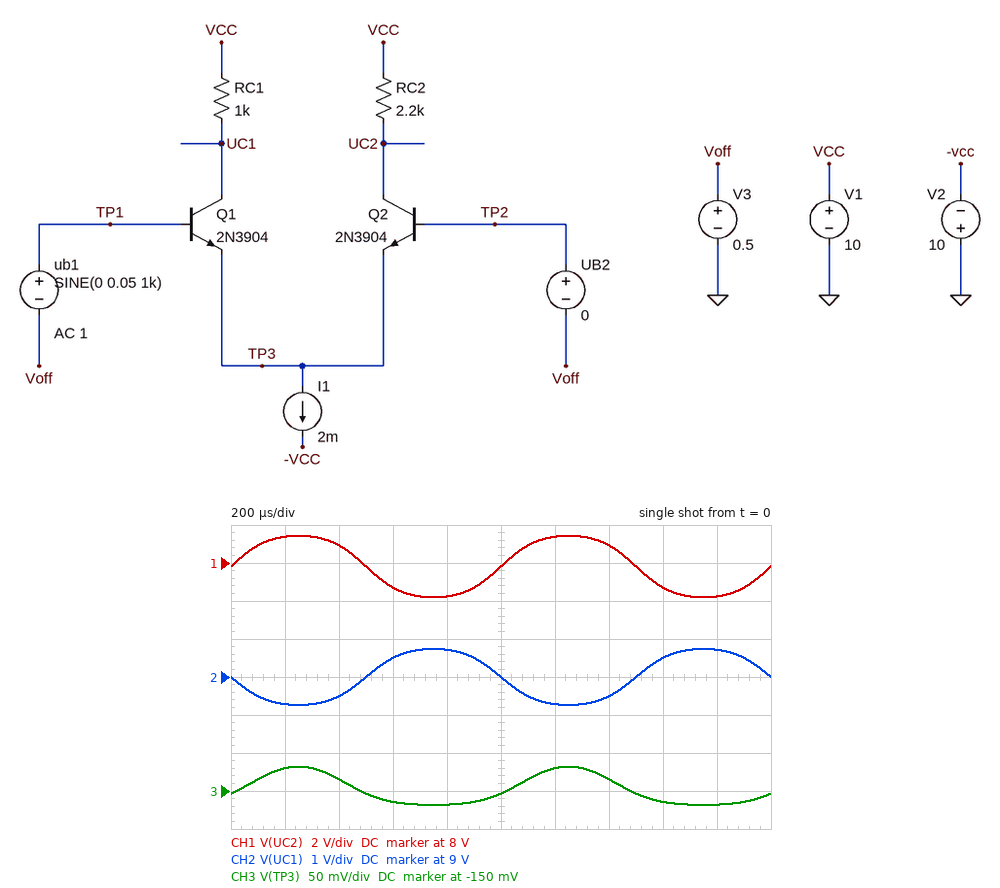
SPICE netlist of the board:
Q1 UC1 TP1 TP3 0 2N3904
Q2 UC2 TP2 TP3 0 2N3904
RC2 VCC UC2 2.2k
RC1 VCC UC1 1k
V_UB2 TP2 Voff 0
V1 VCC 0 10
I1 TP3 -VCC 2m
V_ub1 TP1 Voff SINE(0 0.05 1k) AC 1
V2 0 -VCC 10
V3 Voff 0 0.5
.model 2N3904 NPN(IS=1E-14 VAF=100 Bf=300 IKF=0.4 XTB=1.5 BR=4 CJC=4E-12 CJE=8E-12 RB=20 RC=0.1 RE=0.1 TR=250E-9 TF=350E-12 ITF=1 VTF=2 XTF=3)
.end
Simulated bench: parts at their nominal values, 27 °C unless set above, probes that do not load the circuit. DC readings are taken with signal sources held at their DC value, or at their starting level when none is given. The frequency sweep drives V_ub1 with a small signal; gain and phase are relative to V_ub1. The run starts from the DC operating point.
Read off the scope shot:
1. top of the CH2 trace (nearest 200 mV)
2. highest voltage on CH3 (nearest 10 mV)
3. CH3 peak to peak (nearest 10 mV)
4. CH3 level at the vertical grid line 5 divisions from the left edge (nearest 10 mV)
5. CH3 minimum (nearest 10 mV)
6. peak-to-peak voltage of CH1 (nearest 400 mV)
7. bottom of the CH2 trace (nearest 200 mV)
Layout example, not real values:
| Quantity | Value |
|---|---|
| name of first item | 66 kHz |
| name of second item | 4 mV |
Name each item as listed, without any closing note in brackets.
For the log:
| Quantity | Value |
|---|---|
| top of the CH2 trace | 9.8 V |
| highest voltage on CH3 | -120 mV |
| CH3 peak to peak | 50 mV |
| CH3 level at the vertical grid line 5 divisions from the left edge | -150 mV |
| CH3 minimum | -170 mV |
| peak-to-peak voltage of CH1 | 3.2 V |
| bottom of the CH2 trace | 8.2 V |
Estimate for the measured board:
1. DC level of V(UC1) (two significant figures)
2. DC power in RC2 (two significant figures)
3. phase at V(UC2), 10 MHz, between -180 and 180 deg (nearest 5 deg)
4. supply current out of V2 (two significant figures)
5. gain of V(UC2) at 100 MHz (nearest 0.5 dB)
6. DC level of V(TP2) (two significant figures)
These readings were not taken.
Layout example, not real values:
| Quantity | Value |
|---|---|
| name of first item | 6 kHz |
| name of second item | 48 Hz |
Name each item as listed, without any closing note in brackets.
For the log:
| Quantity | Value |
|---|---|
| DC level of V(UC1) | 9.0 V |
| DC power in RC2 | 2.2 mW |
| phase at V(UC2), 10 MHz, between -180 and 180 deg | -25 deg |
| supply current out of V2 | 2.0 mA |
| gain of V(UC2) at 100 MHz | 19.0 dB |
| DC level of V(TP2) | 500 mV |
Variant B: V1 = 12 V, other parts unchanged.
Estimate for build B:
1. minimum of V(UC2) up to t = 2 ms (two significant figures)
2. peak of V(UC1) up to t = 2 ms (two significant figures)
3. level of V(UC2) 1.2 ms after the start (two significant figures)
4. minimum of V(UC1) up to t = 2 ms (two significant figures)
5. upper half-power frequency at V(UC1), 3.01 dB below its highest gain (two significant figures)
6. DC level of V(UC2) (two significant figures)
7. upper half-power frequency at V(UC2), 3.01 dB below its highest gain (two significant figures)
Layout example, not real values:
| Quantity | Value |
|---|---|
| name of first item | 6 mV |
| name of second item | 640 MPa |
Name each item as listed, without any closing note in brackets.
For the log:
| Quantity | Value |
|---|---|
| minimum of V(UC2) up to t = 2 ms | 8.2 V |
| peak of V(UC1) up to t = 2 ms | 12 V |
| level of V(UC2) 1.2 ms after the start | 11 V |
| minimum of V(UC1) up to t = 2 ms | 10 V |
| upper half-power frequency at V(UC1), 3.01 dB below its highest gain | 41 MHz |
| DC level of V(UC2) | 9.8 V |
| upper half-power frequency at V(UC2), 3.01 dB below its highest gain | 27 MHz |
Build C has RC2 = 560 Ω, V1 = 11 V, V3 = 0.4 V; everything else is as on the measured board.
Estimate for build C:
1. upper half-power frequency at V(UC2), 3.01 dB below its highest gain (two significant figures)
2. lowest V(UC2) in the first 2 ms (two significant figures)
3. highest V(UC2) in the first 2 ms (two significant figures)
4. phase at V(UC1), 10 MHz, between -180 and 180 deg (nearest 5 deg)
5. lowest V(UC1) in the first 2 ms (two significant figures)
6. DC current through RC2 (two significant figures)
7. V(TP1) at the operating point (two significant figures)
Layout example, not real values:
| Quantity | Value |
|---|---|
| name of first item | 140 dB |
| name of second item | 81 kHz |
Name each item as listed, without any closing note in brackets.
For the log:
| Quantity | Value |
|---|---|
| upper half-power frequency at V(UC2), 3.01 dB below its highest gain | 68 MHz |
| lowest V(UC2) in the first 2 ms | 10 V |
| highest V(UC2) in the first 2 ms | 11 V |
| phase at V(UC1), 10 MHz, between -180 and 180 deg | 170 deg |
| lowest V(UC1) in the first 2 ms | 9.3 V |
| DC current through RC2 | 1.0 mA |
| V(TP1) at the operating point | 400 mV |
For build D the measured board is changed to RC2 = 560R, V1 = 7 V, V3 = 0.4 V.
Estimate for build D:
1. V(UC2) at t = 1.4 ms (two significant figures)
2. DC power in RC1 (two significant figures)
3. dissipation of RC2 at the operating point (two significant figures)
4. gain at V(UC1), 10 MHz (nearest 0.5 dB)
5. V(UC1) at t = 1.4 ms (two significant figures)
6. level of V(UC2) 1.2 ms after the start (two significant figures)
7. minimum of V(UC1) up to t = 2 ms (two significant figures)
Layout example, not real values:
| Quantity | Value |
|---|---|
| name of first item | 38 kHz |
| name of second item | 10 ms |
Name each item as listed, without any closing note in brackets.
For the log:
| Quantity | Value |
|---|---|
| V(UC2) at t = 1.4 ms | 6.7 V |
| DC power in RC1 | 990 µW |
| dissipation of RC2 at the operating point | 560 µW |
| gain at V(UC1), 10 MHz | 25.5 dB |
| V(UC1) at t = 1.4 ms | 5.5 V |
| level of V(UC2) 1.2 ms after the start | 6.8 V |
| minimum of V(UC1) up to t = 2 ms | 5.3 V |
